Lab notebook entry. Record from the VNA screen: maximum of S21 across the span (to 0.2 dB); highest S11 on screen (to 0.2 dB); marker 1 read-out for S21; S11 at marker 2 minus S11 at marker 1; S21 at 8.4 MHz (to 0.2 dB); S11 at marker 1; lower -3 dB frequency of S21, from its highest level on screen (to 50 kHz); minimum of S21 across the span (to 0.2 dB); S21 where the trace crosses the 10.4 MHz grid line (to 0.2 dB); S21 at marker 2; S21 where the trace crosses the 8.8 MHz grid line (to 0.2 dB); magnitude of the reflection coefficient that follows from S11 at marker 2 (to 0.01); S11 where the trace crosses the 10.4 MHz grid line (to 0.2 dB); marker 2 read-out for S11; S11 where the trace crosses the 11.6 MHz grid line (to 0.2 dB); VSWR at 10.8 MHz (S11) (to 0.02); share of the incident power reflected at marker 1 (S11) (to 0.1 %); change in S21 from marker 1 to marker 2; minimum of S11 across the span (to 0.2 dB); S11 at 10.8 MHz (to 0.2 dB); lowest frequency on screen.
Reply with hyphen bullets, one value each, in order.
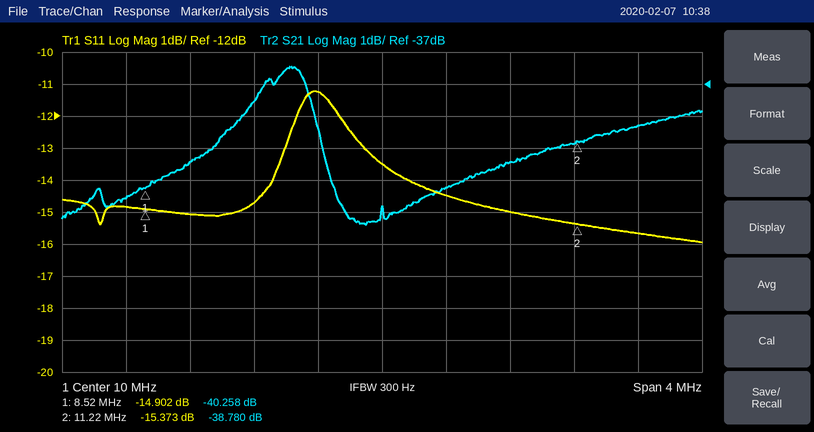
- -36.4 dB
- -11.2 dB
- -40.258 dB
- -0.471 dB
- -40.6 dB
- -14.902 dB
- 8.80 MHz
- -41.4 dB
- -40.2 dB
- -38.780 dB
- -39.4 dB
- 0.17
- -14.4 dB
- -15.373 dB
- -15.6 dB
- 1.44
- 3.2 %
- 1.478 dB
- -16.0 dB
- -15.0 dB
- 8 MHz
